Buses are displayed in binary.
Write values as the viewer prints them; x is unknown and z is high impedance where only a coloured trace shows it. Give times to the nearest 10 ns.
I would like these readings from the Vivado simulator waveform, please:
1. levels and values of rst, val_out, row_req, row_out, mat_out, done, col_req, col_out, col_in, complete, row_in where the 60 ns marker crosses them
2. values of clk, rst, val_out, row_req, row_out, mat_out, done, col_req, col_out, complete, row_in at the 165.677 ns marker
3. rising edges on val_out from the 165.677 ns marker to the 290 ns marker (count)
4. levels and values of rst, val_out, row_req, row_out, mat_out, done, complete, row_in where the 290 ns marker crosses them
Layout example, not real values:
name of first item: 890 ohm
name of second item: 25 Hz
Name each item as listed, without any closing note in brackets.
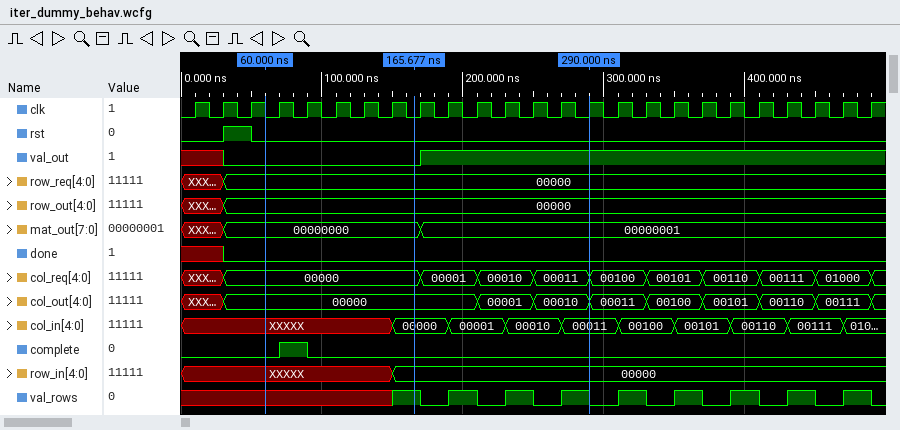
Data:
levels and values of rst, val_out, row_req, row_out, mat_out, done, col_req, col_out, col_in, complete, row_in where the 60 ns marker crosses them: rst=0, val_out=0, row_req=00000, row_out=00000, mat_out=00000000, done=0, col_req=00000, col_out=00000, col_in=XXXXX, complete=0, row_in=XXXXX
values of clk, rst, val_out, row_req, row_out, mat_out, done, col_req, col_out, complete, row_in at the 165.677 ns marker: clk=0, rst=0, val_out=0, row_req=00000, row_out=00000, mat_out=00000000, done=0, col_req=00000, col_out=00000, complete=0, row_in=00000
rising edges on val_out from the 165.677 ns marker to the 290 ns marker: 1
levels and values of rst, val_out, row_req, row_out, mat_out, done, complete, row_in where the 290 ns marker crosses them: rst=0, val_out=1, row_req=00000, row_out=00000, mat_out=00000001, done=0, complete=0, row_in=00000
